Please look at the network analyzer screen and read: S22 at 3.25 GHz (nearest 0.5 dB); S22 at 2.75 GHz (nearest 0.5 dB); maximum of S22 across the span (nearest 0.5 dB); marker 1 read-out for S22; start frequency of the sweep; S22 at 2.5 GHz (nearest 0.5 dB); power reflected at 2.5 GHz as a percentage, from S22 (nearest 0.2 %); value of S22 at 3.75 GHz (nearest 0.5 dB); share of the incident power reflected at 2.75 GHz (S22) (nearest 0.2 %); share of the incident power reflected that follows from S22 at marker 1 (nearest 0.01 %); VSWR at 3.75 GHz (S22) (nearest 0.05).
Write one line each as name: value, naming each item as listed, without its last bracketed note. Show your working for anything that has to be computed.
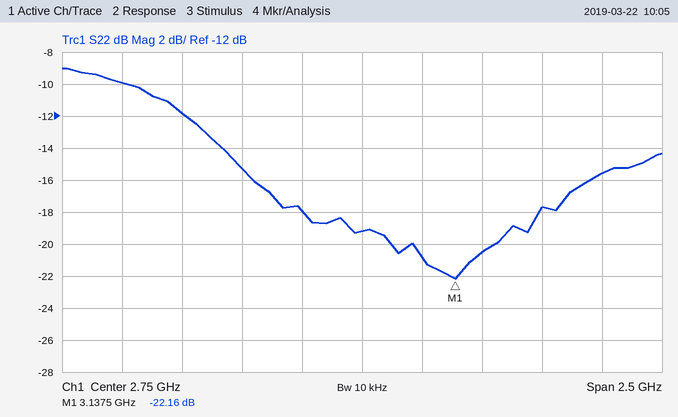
S22 at 3.25 GHz: -20.5 dB
S22 at 2.75 GHz: -19.0 dB
maximum of S22 across the span: -9.0 dB
marker 1 read-out for S22: -22.16 dB
start frequency of the sweep: 1.5 GHz
S22 at 2.5 GHz: -18.0 dB
power reflected at 2.5 GHz as a percentage, from S22: 10^(-18/10) ≈ 1.6 %
value of S22 at 3.75 GHz: -15.5 dB
share of the incident power reflected at 2.75 GHz (S22): 10^(-19/10) ≈ 1.26 %, so 1.2 % to the nearest 0.2 %
share of the incident power reflected that follows from S22 at marker 1: 10^(-22.16/10) ≈ 0.61 %
VSWR at 3.75 GHz (S22): |Γ| = 10^(-15.5/20) = 0.1679; VSWR = (1 + 0.1679)/(1 − 0.1679) ≈ 1.40
